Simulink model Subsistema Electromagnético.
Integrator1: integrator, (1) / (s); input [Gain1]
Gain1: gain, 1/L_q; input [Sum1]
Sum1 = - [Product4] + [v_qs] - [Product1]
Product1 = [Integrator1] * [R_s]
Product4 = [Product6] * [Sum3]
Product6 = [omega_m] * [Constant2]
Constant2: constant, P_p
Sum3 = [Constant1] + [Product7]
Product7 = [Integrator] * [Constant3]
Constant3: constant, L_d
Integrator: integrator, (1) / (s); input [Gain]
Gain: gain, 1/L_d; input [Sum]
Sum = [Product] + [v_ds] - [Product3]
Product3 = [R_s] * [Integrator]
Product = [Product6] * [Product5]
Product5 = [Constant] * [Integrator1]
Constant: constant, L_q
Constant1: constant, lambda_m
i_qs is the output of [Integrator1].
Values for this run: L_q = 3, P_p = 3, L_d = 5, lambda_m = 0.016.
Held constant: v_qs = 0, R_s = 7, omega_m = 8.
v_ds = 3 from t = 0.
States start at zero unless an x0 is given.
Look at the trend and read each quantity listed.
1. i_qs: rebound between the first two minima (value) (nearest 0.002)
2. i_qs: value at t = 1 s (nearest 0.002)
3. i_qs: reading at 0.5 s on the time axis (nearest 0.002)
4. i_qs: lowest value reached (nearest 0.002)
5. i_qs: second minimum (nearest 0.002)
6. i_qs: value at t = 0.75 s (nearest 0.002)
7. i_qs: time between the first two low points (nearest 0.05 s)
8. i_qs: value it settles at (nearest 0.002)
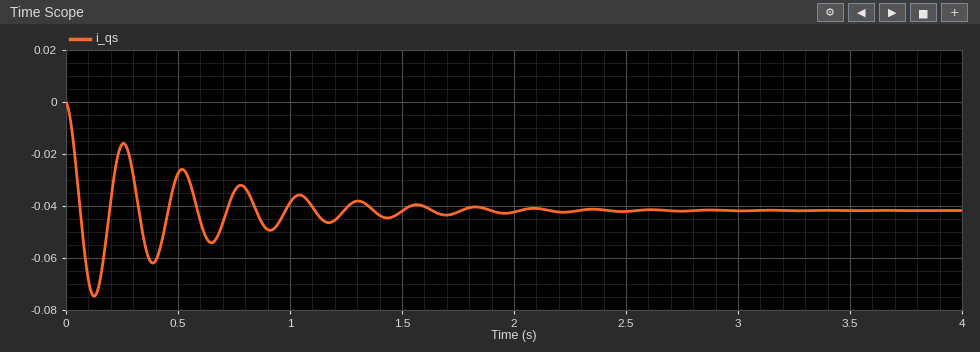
-0.016
-0.038
-0.028
-0.074
-0.062
-0.034
0.25 s
-0.042
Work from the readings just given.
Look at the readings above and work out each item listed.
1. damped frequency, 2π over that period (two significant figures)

25 rad/s
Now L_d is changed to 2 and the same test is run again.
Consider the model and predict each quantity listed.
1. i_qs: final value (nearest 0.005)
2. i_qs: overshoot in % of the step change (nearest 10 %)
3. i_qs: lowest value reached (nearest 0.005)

-0.040
70 %
-0.070
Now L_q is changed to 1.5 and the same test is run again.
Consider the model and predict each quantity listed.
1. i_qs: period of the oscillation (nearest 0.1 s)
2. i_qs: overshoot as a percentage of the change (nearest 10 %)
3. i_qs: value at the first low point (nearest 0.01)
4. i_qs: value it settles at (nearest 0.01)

0.3 s
70 %
-0.14
-0.08
